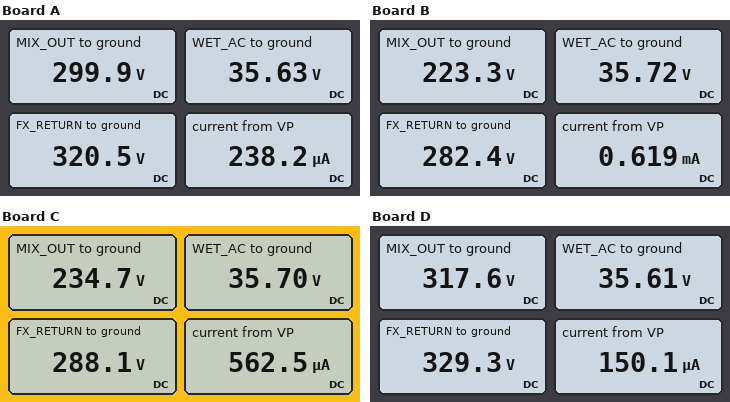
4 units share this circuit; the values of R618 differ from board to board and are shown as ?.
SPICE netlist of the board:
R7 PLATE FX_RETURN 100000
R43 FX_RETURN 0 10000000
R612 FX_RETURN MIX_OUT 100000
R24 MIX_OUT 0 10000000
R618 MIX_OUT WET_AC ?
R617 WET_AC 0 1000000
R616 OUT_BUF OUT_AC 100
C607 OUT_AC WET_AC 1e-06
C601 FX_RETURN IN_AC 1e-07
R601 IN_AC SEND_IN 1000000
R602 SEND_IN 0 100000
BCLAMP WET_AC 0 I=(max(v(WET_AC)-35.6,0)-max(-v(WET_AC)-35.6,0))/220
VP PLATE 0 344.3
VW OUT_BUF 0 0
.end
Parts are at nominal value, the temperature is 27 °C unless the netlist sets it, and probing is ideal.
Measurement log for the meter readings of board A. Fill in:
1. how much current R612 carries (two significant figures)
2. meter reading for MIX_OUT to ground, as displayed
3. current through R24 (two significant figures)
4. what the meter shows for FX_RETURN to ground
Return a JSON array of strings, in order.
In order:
["210 µA", "299.9 V", "30 µA", "320.5 V"]
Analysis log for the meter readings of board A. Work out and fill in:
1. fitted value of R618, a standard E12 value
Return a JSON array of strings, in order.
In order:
["1.5 MΩ"]
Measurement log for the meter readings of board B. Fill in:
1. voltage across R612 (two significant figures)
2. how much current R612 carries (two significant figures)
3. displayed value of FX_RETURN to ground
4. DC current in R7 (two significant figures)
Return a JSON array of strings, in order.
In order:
["59 V", "590 µA", "282.4 V", "620 µA"]
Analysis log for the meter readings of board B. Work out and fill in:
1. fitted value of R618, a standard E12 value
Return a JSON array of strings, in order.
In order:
["330 kΩ"]
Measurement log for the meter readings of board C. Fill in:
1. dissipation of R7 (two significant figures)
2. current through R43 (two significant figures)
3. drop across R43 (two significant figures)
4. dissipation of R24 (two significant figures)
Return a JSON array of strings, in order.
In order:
["32 mW", "29 µA", "290 V", "5.5 mW"]
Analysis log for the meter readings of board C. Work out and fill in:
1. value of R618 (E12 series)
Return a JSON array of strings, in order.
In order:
["390 kΩ"]
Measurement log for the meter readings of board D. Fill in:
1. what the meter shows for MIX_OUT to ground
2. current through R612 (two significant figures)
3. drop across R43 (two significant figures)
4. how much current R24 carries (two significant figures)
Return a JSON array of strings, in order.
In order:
["317.6 V", "120 µA", "330 V", "32 µA"]
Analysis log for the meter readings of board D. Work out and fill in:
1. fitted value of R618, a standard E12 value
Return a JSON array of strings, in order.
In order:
["3.3 MΩ"]
